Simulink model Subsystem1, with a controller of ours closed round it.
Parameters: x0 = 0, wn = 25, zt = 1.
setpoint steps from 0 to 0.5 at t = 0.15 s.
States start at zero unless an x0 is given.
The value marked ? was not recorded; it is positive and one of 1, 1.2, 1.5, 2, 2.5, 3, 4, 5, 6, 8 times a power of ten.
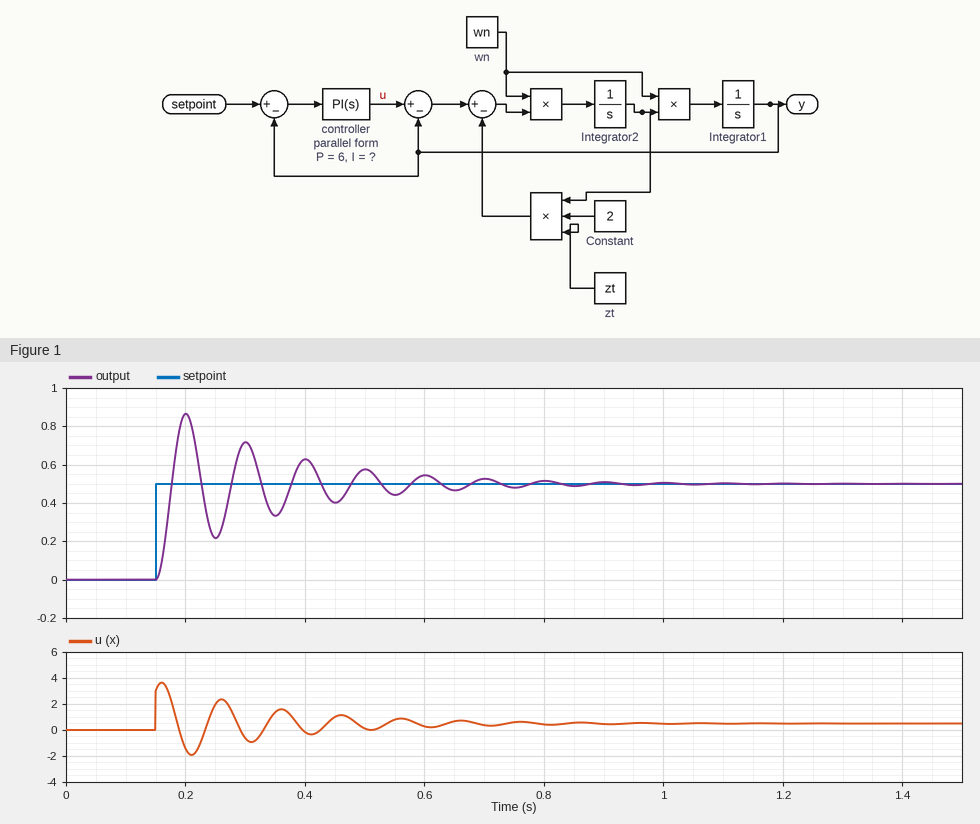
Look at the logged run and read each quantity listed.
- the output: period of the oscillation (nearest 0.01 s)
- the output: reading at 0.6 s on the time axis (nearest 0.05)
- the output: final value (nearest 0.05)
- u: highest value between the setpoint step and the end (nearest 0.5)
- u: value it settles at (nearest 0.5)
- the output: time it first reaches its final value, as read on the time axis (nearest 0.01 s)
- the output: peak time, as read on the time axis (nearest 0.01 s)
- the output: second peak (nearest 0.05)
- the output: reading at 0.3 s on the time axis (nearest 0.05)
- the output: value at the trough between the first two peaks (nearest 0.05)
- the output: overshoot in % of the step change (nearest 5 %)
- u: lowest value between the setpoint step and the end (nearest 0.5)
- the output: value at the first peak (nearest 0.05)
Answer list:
0.10 s
0.55
0.50
3.5
0.5
0.18 s
0.20 s
0.70
0.70
0.20
75 %
-2.0
0.85
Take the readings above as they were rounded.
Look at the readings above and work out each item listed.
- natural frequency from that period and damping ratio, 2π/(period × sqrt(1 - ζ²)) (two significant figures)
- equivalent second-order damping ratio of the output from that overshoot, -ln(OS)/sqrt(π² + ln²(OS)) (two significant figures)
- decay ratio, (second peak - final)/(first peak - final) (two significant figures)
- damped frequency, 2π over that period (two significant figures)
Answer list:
63 rad/s
0.091
0.57
63 rad/s
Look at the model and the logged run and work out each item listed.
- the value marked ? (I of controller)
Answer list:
250
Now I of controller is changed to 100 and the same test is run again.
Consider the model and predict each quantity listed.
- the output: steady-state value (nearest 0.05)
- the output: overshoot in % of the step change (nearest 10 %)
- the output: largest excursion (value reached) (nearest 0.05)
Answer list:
0.50
40 %
0.70
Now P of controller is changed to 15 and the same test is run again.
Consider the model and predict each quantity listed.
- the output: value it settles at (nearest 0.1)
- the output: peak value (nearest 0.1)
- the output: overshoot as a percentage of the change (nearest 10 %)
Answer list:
0.5
0.8
60 %
